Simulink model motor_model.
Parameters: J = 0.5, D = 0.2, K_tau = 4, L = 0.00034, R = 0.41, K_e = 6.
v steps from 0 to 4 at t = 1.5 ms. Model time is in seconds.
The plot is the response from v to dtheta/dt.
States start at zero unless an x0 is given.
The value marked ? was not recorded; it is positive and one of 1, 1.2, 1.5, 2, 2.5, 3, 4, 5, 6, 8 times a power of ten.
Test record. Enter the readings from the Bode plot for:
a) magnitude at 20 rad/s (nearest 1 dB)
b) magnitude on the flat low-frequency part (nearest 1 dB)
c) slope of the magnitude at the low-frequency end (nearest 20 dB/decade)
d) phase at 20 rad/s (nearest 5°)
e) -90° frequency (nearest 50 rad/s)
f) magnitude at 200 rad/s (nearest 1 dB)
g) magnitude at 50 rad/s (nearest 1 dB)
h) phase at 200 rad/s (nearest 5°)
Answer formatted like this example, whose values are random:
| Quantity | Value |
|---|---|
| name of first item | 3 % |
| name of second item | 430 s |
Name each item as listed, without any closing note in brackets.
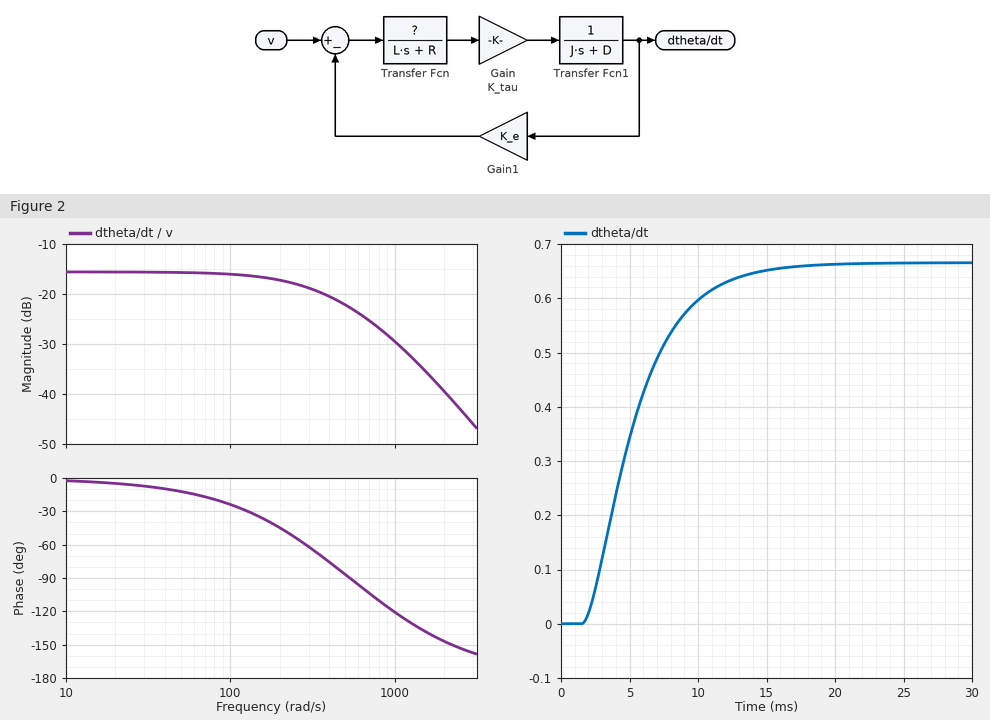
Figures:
| Quantity | Value |
|---|---|
| magnitude at 20 rad/s | -16 dB |
| magnitude on the flat low-frequency part | -16 dB |
| slope of the magnitude at the low-frequency end | 0 dB/decade |
| phase at 20 rad/s | -5° |
| -90° frequency | 550 rad/s |
| magnitude at 200 rad/s | -17 dB |
| magnitude at 50 rad/s | -16 dB |
| phase at 200 rad/s | -45° |
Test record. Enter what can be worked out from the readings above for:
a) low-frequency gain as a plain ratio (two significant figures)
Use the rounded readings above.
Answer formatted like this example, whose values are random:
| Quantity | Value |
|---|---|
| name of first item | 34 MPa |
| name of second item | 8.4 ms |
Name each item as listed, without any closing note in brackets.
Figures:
| Quantity | Value |
|---|---|
| low-frequency gain as a plain ratio | 0.16 |
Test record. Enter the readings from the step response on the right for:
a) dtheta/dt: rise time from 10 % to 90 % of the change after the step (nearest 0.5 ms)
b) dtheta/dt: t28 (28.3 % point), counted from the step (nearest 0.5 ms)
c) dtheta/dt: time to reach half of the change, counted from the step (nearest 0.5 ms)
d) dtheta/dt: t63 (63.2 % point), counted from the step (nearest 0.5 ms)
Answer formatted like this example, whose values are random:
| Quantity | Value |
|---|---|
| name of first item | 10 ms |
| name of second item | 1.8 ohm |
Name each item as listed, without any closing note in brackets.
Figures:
| Quantity | Value |
|---|---|
| dtheta/dt: rise time from 10 % to 90 % of the change after the step | 7.5 ms |
| dtheta/dt: t28 (28.3 % point), counted from the step | 2.0 ms |
| dtheta/dt: time to reach half of the change, counted from the step | 3.5 ms |
| dtheta/dt: t63 (63.2 % point), counted from the step | 4.5 ms |
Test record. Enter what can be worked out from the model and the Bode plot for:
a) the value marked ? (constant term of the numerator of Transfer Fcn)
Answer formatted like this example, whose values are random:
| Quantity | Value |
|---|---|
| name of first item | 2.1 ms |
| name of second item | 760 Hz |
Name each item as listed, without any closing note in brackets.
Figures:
| Quantity | Value |
|---|---|
| the value marked ? | 2 |
